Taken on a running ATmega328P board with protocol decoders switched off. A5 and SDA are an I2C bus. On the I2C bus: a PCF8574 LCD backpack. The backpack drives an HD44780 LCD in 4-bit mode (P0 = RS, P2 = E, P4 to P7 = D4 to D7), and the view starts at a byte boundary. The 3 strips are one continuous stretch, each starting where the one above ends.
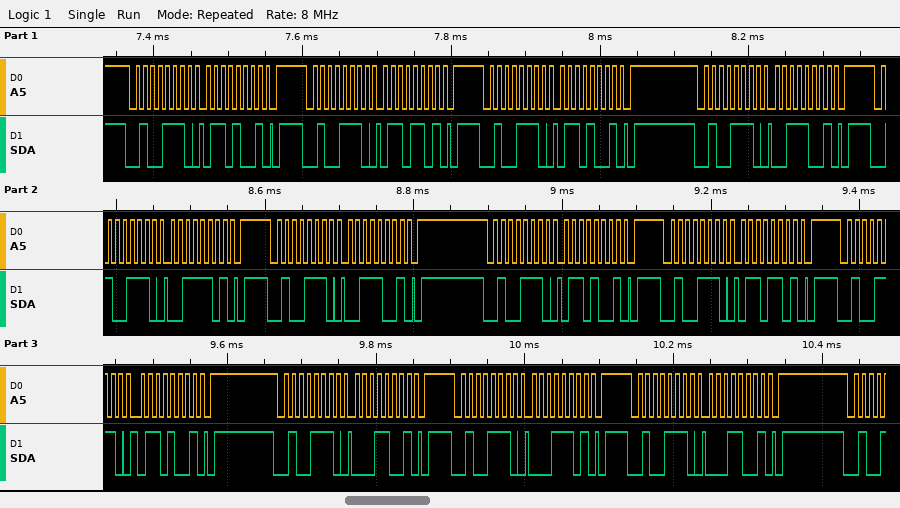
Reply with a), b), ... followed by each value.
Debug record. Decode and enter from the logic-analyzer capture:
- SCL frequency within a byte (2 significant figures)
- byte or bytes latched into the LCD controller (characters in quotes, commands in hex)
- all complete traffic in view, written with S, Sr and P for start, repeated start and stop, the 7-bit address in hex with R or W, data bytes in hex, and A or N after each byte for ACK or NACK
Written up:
a) 100 kHz
b) 'c' 'a'
c) S 27W A 69 A P S 27W A 6D A P S 27W A 69 A P S 27W A 39 A P S 27W A 3D A P S 27W A 39 A P S 27W A 69 A P S 27W A 6D A P S 27W A 69 A P S 27W A 19 A P S 27W A 1D A P S 27W A 19 A P
